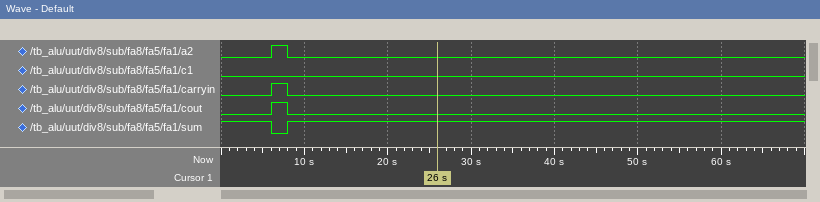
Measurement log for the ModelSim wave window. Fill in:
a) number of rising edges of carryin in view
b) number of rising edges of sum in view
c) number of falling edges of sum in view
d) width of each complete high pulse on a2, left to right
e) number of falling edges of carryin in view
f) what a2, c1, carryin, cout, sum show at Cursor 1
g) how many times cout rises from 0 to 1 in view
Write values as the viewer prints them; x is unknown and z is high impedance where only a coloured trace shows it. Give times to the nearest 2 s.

1
1
1
2 s
1
a2=0, c1=0, carryin=0, cout=0, sum=1
1
